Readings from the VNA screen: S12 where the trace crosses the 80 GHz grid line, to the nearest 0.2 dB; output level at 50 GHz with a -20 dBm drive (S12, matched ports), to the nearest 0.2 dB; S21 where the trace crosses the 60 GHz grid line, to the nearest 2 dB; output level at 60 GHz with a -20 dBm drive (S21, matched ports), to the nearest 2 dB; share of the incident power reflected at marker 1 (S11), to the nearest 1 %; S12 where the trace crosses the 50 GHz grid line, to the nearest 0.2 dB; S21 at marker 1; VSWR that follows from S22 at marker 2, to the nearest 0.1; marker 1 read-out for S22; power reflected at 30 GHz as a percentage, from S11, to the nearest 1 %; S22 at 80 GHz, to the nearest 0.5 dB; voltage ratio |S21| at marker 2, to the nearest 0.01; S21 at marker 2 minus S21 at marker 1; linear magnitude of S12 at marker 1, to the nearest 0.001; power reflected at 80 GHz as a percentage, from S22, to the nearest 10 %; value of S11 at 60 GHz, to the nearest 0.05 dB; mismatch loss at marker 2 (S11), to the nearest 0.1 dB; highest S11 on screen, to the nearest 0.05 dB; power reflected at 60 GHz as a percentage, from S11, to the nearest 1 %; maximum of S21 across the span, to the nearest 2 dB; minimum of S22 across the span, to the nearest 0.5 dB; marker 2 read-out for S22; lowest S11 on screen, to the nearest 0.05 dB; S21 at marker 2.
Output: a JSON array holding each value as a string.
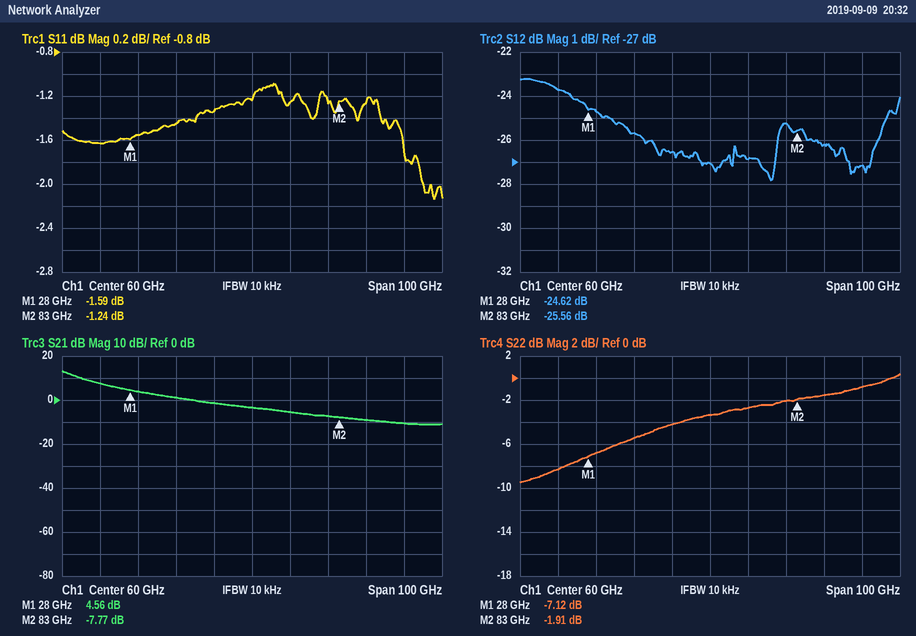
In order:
["-25.2 dB", "-46.6 dBm", "-4 dB", "-24 dBm", "69 %", "-26.6 dB", "4.56 dB", "9.1", "-7.12 dB", "70 %", "-2.0 dB", "0.41", "-12.33 dB", "0.059", "60 %", "-1.25 dB", "6.0 dB", "-1.10 dB", "75 %", "14 dB", "-9.5 dB", "-1.91 dB", "-2.15 dB", "-7.77 dB"]
